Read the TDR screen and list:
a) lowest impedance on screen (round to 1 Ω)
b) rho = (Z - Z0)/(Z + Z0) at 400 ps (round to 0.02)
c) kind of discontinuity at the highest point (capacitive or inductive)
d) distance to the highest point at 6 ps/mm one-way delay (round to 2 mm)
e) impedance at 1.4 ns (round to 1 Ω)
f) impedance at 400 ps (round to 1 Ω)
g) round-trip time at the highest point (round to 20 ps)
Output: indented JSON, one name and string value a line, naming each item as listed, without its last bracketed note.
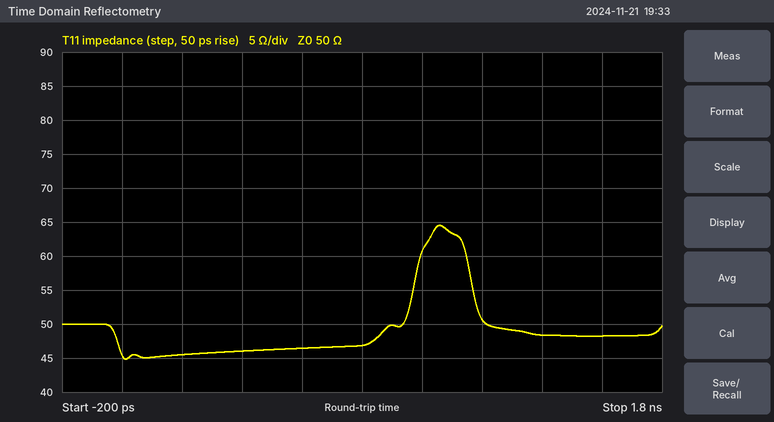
{
  "lowest impedance on screen": "45 Ω",
  "rho = (Z - Z0)/(Z + Z0) at 400 ps": "-0.04",
  "kind of discontinuity at the highest point": "inductive",
  "distance to the highest point at 6 ps/mm one-way delay": "88 mm",
  "impedance at 1.4 ns": "48 Ω",
  "impedance at 400 ps": "46 Ω",
  "round-trip time at the highest point": "1.06 ns"
}
